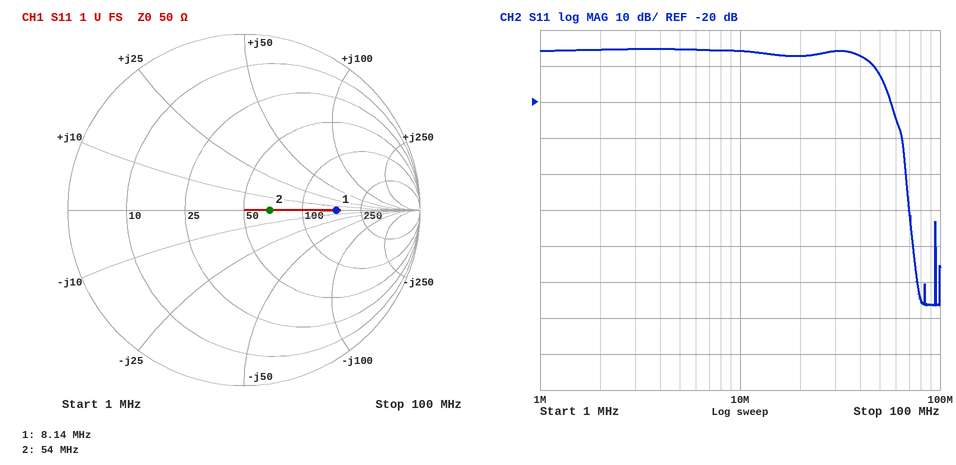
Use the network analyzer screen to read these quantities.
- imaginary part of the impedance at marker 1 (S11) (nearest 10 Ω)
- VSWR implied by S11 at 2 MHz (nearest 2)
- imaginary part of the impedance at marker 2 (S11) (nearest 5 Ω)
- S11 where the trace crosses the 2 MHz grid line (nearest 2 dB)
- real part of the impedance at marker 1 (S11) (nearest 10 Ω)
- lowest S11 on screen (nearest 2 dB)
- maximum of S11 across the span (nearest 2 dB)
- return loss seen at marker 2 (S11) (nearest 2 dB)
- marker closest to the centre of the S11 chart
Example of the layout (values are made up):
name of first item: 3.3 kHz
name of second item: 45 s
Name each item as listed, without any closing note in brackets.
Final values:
imaginary part of the impedance at marker 1 (S11): 0 Ω
VSWR implied by S11 at 2 MHz: 4
imaginary part of the impedance at marker 2 (S11): 0 Ω
S11 where the trace crosses the 2 MHz grid line: -6 dB
real part of the impedance at marker 1 (S11): 160 Ω
lowest S11 on screen: -76 dB
maximum of S11 across the span: -6 dB
return loss seen at marker 2 (S11): 16 dB
marker closest to the centre of the S11 chart: marker 2
